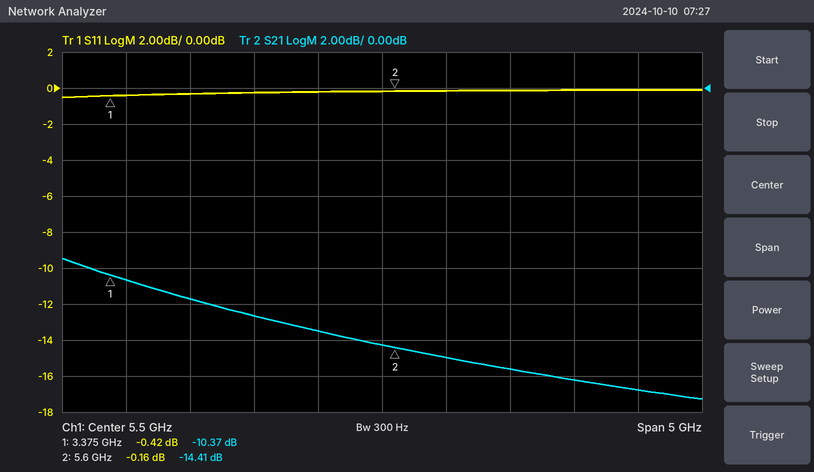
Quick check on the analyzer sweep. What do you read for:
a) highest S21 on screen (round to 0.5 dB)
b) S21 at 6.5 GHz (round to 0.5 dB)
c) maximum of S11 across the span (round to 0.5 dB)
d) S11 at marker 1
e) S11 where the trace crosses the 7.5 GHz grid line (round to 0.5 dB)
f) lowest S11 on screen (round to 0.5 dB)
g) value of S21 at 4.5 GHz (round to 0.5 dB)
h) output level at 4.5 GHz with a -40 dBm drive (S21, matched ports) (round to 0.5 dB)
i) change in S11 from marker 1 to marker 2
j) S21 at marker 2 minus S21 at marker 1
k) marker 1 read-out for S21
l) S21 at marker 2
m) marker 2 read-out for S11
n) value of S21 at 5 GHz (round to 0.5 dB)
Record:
-9.5 dB
-15.5 dB
0.0 dB
-0.42 dB
0.0 dB
-0.5 dB
-12.5 dB
-52.5 dBm
0.26 dB
-4.04 dB
-10.37 dB
-14.41 dB
-0.16 dB
-13.5 dB
